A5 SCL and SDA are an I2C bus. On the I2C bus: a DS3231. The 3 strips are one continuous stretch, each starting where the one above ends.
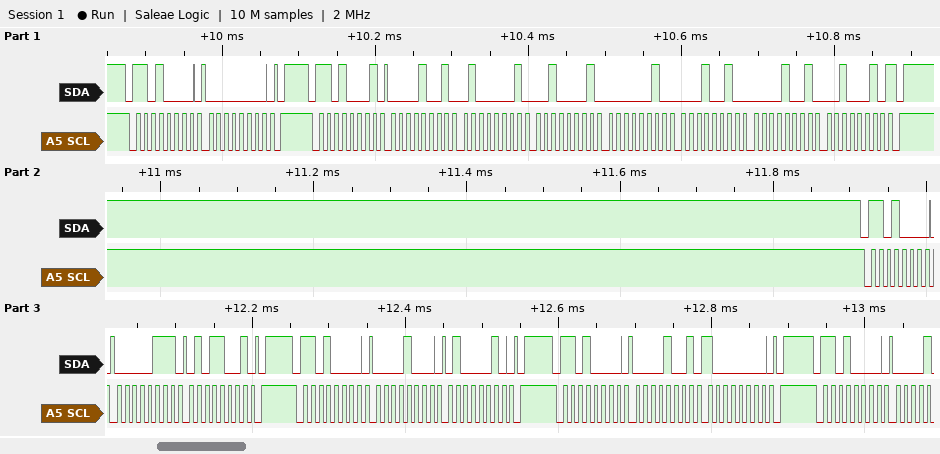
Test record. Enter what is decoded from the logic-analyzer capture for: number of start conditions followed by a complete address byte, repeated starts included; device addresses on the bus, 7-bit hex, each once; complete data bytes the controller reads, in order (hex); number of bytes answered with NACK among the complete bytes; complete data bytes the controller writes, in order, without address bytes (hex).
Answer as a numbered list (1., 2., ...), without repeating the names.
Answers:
1. 6
2. 0x68
3. 09 41 21 02 12 09 22
4. 1
5. 00 07 59 08 42 09 80
